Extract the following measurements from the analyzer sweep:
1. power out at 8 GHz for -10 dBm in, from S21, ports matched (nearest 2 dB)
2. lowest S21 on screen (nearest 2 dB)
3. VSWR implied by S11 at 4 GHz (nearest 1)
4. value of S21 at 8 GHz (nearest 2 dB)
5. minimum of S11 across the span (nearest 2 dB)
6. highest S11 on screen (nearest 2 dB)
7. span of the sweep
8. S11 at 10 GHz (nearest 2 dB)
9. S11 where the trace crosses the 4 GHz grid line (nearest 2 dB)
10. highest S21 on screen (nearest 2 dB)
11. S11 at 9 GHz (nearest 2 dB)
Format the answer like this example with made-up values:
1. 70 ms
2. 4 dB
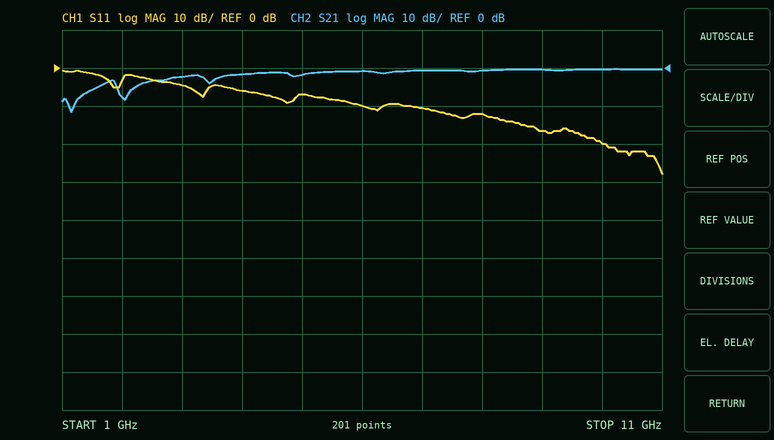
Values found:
1. -10 dBm
2. -12 dB
3. 3
4. 0 dB
5. -28 dB
6. 0 dB
7. 10 GHz
8. -20 dB
9. -6 dB
10. 0 dB
11. -16 dB
